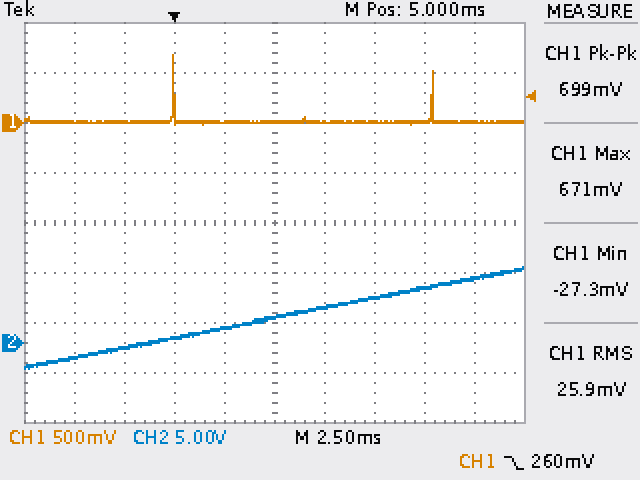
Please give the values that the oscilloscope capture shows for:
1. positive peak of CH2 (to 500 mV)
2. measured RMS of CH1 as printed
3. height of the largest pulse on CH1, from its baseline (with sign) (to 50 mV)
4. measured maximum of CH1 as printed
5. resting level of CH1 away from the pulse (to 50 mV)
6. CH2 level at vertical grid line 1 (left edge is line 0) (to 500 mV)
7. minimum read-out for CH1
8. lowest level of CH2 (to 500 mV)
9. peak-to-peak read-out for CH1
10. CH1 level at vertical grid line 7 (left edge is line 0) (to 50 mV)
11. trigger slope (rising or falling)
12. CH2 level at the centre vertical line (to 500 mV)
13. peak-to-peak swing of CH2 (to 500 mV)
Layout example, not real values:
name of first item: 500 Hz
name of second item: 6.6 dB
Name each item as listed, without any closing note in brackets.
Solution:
positive peak of CH2: 7.5 V
measured RMS of CH1 as printed: 25.9 mV
height of the largest pulse on CH1, from its baseline (with sign): +650 mV
measured maximum of CH1 as printed: 671 mV
resting level of CH1 away from the pulse: 0 mV
CH2 level at vertical grid line 1 (left edge is line 0): -1.5 V
minimum read-out for CH1: -27.3 mV
lowest level of CH2: -2.5 V
peak-to-peak read-out for CH1: 699 mV
CH1 level at vertical grid line 7 (left edge is line 0): 0 mV
trigger slope: falling
CH2 level at the centre vertical line: 2.5 V
peak-to-peak swing of CH2: 10.0 V
